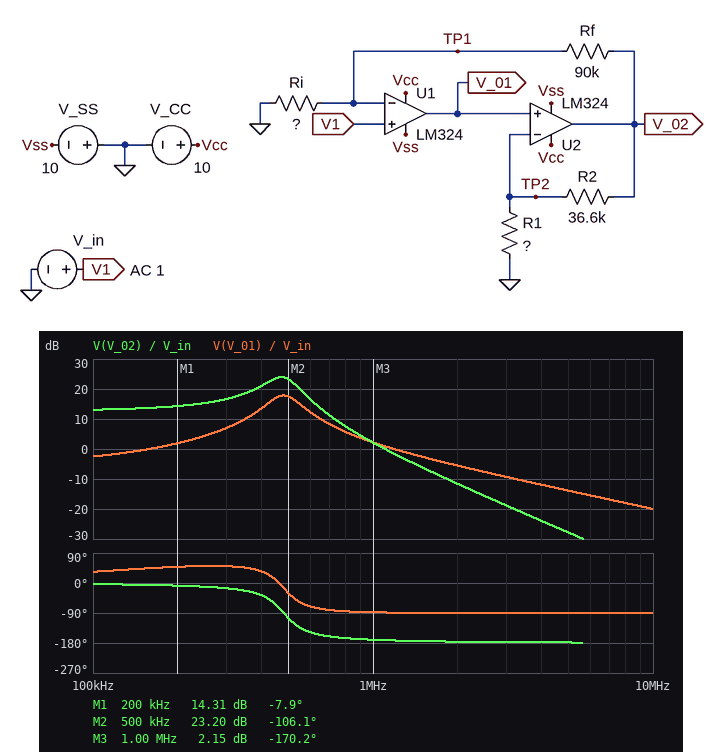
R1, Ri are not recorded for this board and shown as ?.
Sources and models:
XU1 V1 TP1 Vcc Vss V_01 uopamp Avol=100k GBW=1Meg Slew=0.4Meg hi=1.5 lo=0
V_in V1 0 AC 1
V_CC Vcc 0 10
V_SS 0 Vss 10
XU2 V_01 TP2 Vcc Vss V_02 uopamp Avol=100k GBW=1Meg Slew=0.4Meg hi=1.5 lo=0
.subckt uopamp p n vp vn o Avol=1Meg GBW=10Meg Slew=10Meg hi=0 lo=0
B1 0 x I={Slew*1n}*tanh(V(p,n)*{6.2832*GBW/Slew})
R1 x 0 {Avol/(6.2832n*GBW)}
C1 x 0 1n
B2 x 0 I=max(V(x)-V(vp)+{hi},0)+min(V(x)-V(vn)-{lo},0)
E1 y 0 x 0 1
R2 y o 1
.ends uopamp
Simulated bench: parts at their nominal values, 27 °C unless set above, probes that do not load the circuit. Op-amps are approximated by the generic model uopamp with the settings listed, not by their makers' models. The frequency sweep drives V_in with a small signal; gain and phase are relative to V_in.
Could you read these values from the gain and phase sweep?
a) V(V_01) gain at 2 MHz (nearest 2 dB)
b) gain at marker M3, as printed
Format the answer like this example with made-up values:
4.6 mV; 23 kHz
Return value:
-6 dB; 2.15 dB
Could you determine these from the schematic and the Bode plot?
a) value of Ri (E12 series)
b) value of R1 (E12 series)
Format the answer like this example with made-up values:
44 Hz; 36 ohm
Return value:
27 kΩ; 5.6 kΩ
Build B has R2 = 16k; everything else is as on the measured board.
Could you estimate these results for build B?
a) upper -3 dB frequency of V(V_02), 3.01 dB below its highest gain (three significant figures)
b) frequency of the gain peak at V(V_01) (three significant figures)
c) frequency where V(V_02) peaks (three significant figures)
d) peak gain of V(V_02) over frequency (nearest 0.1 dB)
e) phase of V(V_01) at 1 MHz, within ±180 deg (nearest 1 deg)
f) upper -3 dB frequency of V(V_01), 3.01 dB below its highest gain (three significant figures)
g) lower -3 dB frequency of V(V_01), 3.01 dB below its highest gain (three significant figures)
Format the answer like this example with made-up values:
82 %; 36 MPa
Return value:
563 kHz; 472 kHz; 444 kHz; 18.4 dB; -86 deg; 612 kHz; 352 kHz
